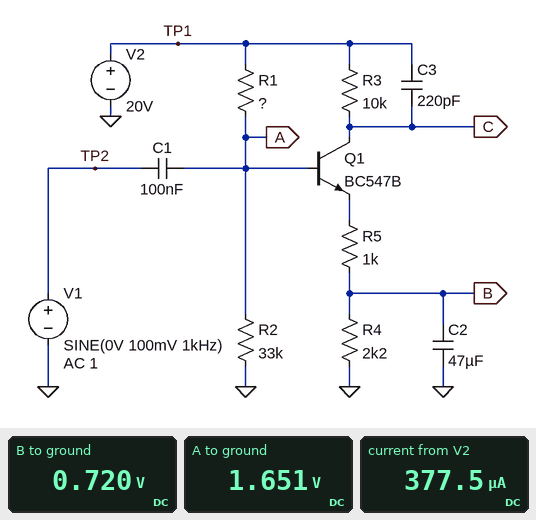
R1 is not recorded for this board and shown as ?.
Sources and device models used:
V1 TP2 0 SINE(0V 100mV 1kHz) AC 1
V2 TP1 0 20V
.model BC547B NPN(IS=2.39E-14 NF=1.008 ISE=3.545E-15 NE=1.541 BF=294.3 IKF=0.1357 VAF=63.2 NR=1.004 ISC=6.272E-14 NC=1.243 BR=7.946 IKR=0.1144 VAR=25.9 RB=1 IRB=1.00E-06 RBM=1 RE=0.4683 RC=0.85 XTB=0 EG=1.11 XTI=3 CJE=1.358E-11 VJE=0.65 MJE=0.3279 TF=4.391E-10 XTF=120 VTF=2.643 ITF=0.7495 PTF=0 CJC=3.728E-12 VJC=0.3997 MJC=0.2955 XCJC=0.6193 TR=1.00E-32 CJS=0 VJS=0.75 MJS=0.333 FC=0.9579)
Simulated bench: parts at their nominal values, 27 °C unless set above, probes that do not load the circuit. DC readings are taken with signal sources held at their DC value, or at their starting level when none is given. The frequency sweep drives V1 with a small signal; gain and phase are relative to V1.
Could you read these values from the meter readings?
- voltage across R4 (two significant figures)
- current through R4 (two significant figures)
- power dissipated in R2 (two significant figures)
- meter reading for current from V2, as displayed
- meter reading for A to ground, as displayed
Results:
720 mV
330 µA
83 µW
377.5 µA
1.651 V
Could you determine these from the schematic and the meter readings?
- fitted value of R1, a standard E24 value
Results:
360 kΩ
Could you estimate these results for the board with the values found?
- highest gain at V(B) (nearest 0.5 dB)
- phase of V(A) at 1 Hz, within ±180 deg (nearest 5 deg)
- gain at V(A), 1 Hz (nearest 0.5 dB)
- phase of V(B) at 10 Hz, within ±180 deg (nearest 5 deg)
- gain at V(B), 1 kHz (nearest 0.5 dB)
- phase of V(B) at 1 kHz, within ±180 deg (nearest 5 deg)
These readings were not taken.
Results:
-26.0 dB
90 deg
-34.5 dB
15 deg
-50.0 dB
-85 deg
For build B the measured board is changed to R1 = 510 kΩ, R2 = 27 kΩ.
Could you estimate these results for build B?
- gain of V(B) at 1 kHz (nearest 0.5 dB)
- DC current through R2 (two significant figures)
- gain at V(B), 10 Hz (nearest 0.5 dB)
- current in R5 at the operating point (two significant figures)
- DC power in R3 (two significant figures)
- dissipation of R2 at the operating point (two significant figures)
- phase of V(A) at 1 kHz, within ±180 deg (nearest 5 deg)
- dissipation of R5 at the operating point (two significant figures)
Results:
-51.0 dB
37 µA
-28.0 dB
130 µA
170 µW
37 µW
5 deg
17 µW
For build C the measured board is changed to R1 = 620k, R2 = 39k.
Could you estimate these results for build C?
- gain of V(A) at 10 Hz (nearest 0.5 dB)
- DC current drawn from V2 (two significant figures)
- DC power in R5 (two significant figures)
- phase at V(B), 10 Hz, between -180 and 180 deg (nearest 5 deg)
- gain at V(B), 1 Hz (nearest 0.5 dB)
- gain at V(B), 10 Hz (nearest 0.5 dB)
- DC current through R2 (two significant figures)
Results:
-13.5 dB
210 µA
33 µW
10 deg
-37.0 dB
-25.0 dB
30 µA
